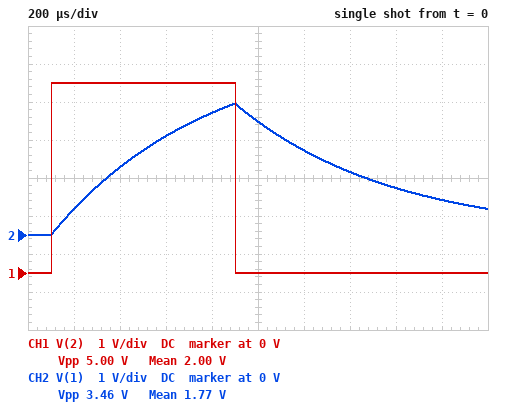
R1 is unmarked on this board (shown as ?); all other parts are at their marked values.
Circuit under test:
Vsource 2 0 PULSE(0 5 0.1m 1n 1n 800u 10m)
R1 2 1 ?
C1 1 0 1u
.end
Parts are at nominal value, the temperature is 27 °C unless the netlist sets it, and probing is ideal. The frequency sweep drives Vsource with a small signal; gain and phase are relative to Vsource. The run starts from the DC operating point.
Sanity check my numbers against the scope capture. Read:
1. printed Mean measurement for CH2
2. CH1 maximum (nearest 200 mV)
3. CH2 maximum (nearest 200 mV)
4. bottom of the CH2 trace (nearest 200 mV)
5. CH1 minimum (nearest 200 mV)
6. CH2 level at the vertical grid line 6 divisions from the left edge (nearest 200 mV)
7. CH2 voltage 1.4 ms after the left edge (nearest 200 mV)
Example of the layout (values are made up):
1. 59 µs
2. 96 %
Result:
1. 1.77 V
2. 5.0 V
3. 3.4 V
4. 0 V
5. 0 V
6. 2.2 V
7. 1.6 V
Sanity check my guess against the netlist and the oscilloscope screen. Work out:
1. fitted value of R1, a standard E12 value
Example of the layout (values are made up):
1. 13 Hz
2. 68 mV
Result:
1. 680 Ω
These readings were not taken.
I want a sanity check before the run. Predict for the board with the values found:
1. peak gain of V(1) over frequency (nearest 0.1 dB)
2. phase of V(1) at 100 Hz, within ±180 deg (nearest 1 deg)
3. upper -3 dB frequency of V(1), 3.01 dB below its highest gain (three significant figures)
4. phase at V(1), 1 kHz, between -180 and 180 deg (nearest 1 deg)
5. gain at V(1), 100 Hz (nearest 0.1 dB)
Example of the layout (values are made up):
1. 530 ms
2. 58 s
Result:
1. 0 dB
2. -23 deg
3. 234 Hz
4. -77 deg
5. -0.7 dB
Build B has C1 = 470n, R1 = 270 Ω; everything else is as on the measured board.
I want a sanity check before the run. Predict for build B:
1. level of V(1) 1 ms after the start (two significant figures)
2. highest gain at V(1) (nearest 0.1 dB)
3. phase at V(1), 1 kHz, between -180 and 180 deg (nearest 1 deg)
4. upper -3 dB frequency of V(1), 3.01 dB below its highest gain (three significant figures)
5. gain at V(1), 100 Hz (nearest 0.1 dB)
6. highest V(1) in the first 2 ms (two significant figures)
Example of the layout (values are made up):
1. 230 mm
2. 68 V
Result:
1. 2.3 V
2. 0 dB
3. -39 deg
4. 1.25 kHz
5. 0 dB
6. 5.0 V
